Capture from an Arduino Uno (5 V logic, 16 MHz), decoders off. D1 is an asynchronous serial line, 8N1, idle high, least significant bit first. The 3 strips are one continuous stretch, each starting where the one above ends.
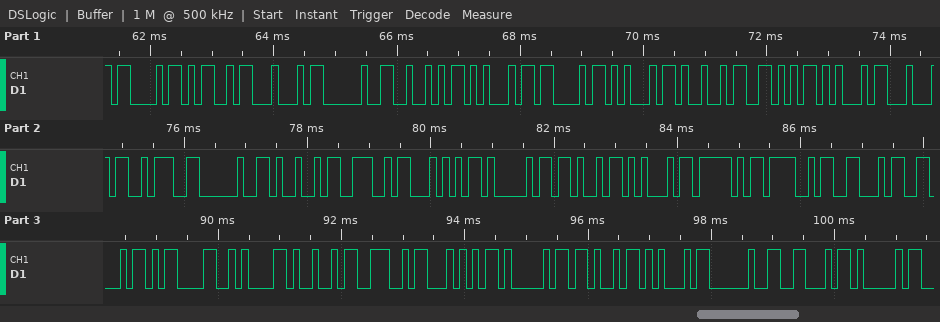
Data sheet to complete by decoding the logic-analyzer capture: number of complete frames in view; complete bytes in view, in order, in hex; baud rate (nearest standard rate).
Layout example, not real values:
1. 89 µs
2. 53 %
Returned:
1. 35
2. 43 4D 44 20 52 45 43 45 49 56 45 44 3A 20 49 4E 54 41 4B 45 5F 4F 46 46 0D 0A 49 4E 54 41 4B 45 20 46 41
3. 9600 baud
